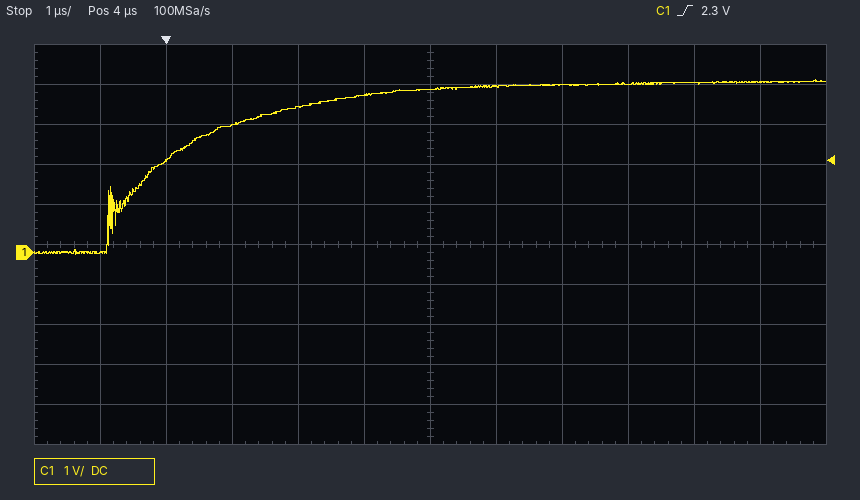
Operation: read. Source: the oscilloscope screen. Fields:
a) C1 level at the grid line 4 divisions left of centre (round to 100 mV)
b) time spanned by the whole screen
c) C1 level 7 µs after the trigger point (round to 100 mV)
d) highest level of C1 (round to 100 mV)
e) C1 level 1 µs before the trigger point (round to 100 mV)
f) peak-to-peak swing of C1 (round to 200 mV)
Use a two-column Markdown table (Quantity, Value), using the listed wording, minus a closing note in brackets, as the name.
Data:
| Quantity | Value |
|---|---|
| C1 level at the grid line 4 divisions left of centre | 2.3 V |
| time spanned by the whole screen | 12 µs |
| C1 level 7 µs after the trigger point | 4.2 V |
| highest level of C1 | 4.3 V |
| C1 level 1 µs before the trigger point | 0.0 V |
| peak-to-peak swing of C1 | 4.4 V |
